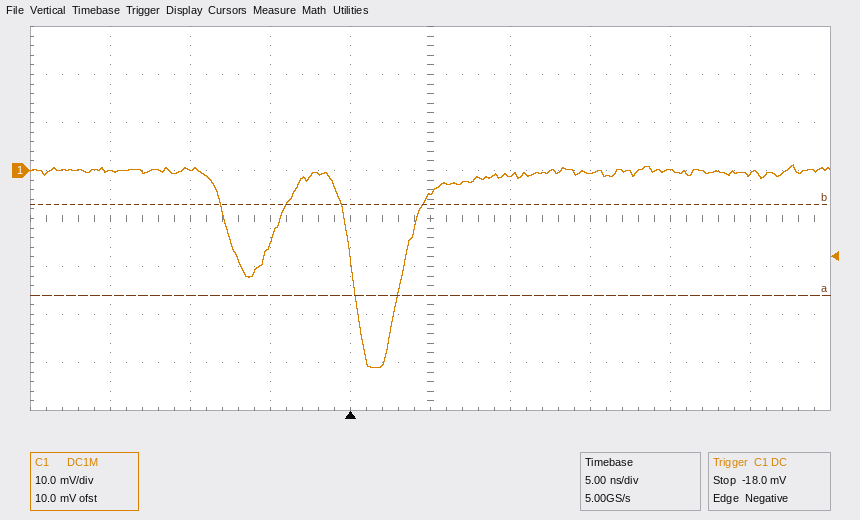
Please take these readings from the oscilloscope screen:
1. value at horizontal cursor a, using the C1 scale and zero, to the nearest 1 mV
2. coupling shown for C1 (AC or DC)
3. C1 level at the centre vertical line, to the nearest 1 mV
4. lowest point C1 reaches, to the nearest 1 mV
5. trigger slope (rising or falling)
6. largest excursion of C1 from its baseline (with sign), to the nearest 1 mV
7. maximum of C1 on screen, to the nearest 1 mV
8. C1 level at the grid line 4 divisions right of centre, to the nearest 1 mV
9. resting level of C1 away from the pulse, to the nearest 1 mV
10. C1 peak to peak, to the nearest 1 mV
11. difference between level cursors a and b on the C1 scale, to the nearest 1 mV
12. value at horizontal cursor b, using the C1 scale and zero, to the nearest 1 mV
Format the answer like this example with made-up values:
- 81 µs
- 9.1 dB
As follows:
- -26 mV
- DC
- -5 mV
- -41 mV
- falling
- -41 mV
- 1 mV
- -1 mV
- 0 mV
- 42 mV
- 19 mV
- -7 mV
